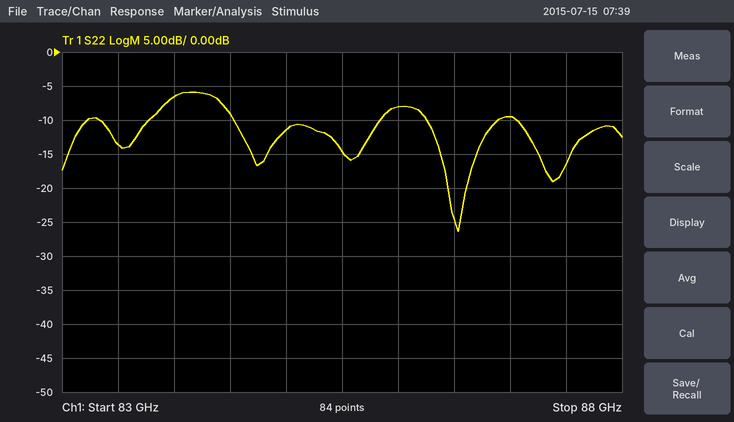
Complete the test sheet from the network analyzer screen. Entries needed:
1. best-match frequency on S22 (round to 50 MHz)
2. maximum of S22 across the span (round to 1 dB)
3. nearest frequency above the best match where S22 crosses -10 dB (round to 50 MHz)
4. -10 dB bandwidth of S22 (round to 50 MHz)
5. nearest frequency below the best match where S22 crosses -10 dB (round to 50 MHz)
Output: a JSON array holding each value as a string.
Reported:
["86.55 GHz", "-6 dB", "86.90 GHz", "650 MHz", "86.25 GHz"]
